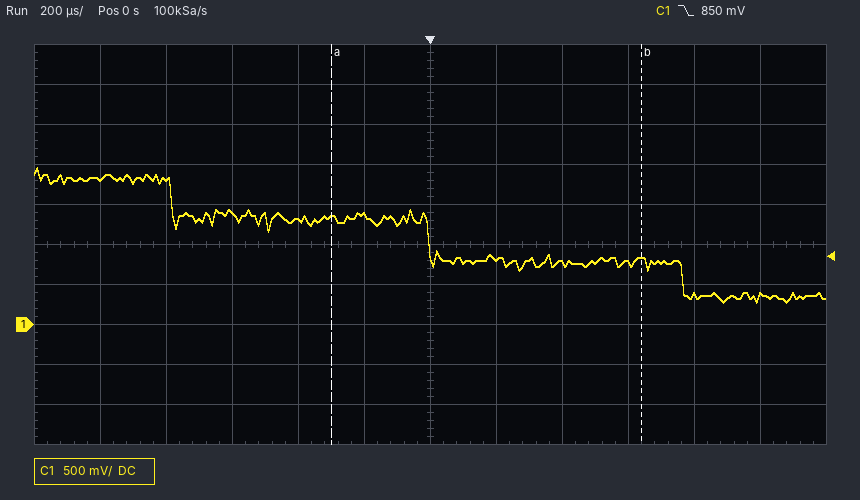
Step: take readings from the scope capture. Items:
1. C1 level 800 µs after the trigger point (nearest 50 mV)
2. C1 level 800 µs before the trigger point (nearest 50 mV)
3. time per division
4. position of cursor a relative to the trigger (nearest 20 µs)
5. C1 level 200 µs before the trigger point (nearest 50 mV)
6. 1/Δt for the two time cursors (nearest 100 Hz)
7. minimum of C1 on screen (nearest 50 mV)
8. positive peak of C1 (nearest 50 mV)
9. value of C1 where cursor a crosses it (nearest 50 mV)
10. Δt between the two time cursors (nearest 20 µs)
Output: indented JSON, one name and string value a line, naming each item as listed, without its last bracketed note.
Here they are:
{
  "C1 level 800 µs after the trigger point": "350 mV",
  "C1 level 800 µs before the trigger point": "1.80 V",
  "time per division": "200 µs",
  "position of cursor a relative to the trigger": "-300 µs",
  "C1 level 200 µs before the trigger point": "1.35 V",
  "1/Δt for the two time cursors": "1.1 kHz",
  "minimum of C1 on screen": "300 mV",
  "positive peak of C1": "1.95 V",
  "value of C1 where cursor a crosses it": "1.35 V",
  "Δt between the two time cursors": "940 µs"
}
